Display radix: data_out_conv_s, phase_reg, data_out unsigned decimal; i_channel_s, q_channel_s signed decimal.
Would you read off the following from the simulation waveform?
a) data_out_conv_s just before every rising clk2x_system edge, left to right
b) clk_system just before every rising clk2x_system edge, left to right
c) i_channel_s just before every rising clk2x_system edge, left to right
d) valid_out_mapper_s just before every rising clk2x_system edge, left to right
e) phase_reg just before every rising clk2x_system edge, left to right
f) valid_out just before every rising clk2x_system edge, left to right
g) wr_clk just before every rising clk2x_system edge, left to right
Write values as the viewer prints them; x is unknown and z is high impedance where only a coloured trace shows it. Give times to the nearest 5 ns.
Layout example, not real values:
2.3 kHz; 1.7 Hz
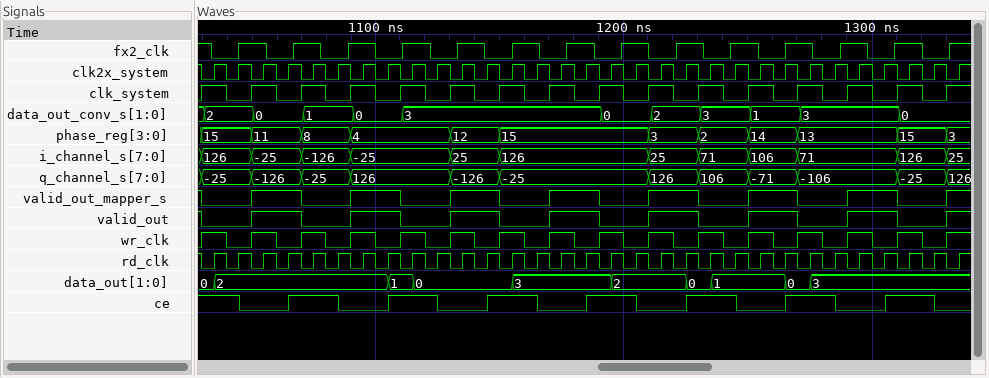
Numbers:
2, 2, 0, 0, 1, 1, 0, 0, 3, 3, 3, 3, 3, 3, 3, 3, 0, 0, 2, 2, 3, 3, 1, 1, 3, 3, 3, 3, 0, 0, 0; 1 0 1 0 1 0 1 0 1 0 1 0 1 0 1 0 1 0 1 0 1 0 1 0 1 0 1 0 1 0 1; 126, 126, -25, -25, -126, -126, -25, -25, -25, -25, 25, 25, 126, 126, 126, 126, 126, 126, 25, 25, 71, 71, 106, 106, 71, 71, 71, 71, 126, 126, 25; 0 0 1 1 0 0 1 1 0 0 1 1 0 0 1 1 0 0 1 1 0 0 1 1 0 0 1 1 0 0 1; 15, 15, 11, 11, 8, 8, 4, 4, 4, 4, 12, 12, 15, 15, 15, 15, 15, 15, 3, 3, 2, 2, 14, 14, 13, 13, 13, 13, 15, 15, 3; 0 0 1 1 0 0 1 1 0 0 1 1 0 0 1 1 0 0 1 1 0 0 1 1 0 0 1 1 0 0 1; 1 0 1 0 1 0 1 0 1 0 1 0 1 0 1 0 1 0 1 0 1 0 1 0 1 0 1 0 1 0 1
